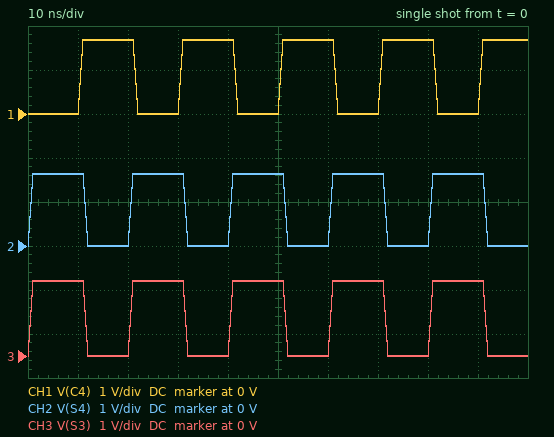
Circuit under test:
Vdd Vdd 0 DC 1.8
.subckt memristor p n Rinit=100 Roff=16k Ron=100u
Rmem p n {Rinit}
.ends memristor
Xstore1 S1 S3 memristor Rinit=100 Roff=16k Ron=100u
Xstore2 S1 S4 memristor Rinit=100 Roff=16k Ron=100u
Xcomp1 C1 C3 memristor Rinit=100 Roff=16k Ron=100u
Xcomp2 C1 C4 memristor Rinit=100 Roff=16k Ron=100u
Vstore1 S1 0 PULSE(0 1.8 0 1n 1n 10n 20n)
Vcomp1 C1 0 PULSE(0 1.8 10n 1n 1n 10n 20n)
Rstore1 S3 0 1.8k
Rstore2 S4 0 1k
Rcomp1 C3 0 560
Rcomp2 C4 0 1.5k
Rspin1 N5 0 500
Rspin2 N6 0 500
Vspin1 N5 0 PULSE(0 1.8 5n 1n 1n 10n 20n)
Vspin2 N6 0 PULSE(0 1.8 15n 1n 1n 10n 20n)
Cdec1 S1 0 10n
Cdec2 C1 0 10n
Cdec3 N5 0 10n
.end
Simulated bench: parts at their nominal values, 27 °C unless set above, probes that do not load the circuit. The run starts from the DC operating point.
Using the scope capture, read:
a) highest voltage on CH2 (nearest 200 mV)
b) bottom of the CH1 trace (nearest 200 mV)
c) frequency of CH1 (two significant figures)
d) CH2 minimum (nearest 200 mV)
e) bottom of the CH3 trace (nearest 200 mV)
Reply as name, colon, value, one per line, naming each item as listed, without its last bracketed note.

highest voltage on CH2: 1.6 V
bottom of the CH1 trace: 0 V
frequency of CH1: 50 MHz
CH2 minimum: 0 V
bottom of the CH3 trace: 0 V
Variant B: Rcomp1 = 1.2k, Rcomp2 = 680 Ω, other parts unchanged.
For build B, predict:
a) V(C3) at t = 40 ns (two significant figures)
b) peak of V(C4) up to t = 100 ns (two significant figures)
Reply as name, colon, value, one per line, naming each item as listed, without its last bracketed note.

V(C3) at t = 40 ns: 1.7 V
peak of V(C4) up to t = 100 ns: 1.6 V
